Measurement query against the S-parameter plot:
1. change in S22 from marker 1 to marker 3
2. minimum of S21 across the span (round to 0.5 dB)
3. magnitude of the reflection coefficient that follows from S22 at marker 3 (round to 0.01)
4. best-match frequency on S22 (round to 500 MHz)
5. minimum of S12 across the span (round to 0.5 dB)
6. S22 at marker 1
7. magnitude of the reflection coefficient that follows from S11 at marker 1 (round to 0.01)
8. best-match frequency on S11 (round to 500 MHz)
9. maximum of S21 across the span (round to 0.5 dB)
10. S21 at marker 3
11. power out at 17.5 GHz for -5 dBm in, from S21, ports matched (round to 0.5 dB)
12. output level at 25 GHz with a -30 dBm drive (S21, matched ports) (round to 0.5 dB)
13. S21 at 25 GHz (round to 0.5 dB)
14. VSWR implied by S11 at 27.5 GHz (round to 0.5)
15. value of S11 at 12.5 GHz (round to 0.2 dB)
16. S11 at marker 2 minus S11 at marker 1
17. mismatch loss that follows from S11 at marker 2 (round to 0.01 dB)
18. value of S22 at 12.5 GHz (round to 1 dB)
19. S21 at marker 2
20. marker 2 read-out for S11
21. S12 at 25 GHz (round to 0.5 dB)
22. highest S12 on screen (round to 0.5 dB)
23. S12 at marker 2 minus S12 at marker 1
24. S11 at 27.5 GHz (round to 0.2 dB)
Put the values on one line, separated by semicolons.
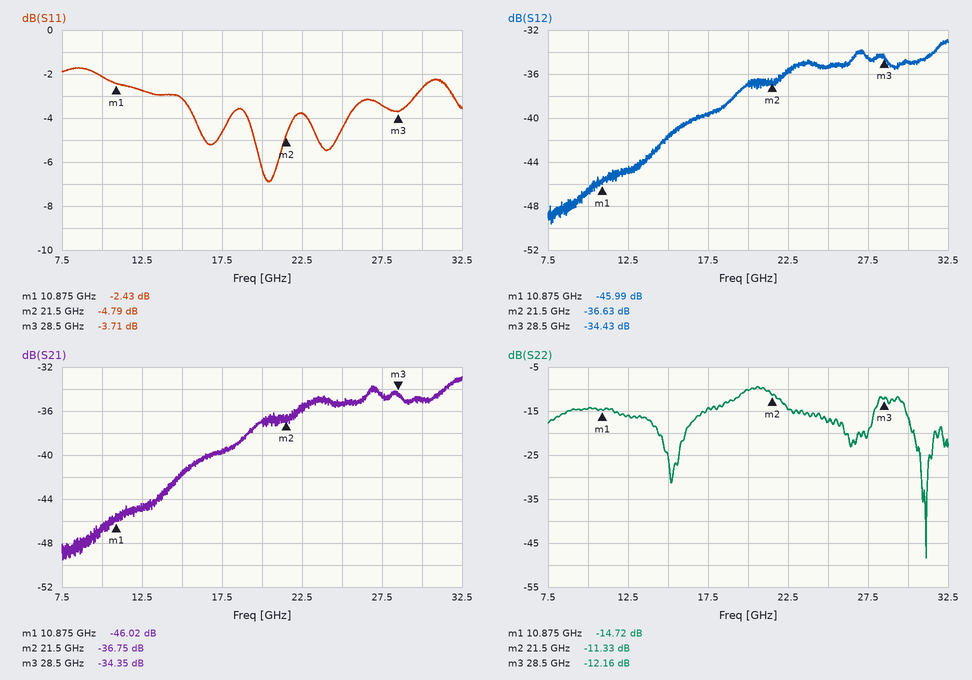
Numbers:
2.56 dB; -49.5 dB; 0.25; 31.0 GHz; -49.5 dB; -14.72 dB; 0.76; 20.5 GHz; -33.0 dB; -34.35 dB; -44.5 dBm; -65.5 dBm; -35.5 dB; 5.0; -2.8 dB; -2.36 dB; 1.75 dB; -16 dB; -36.75 dB; -4.79 dB; -35.5 dB; -33.0 dB; 9.36 dB; -3.4 dB
